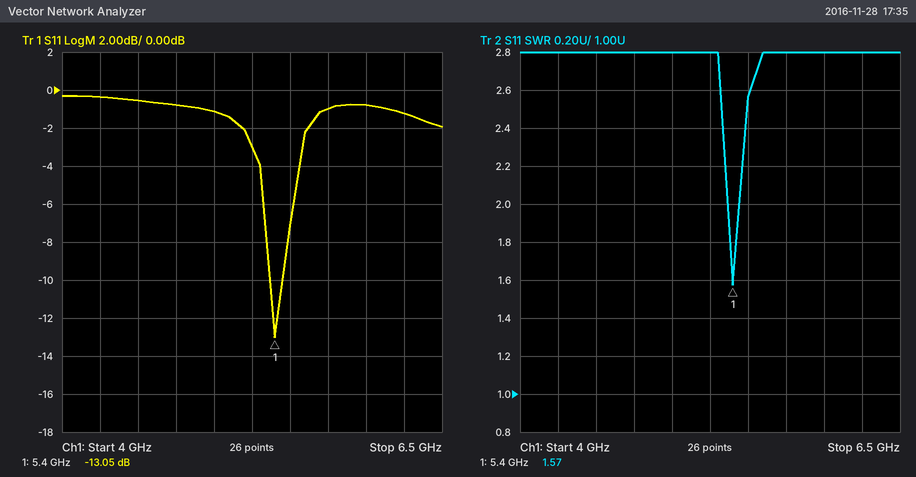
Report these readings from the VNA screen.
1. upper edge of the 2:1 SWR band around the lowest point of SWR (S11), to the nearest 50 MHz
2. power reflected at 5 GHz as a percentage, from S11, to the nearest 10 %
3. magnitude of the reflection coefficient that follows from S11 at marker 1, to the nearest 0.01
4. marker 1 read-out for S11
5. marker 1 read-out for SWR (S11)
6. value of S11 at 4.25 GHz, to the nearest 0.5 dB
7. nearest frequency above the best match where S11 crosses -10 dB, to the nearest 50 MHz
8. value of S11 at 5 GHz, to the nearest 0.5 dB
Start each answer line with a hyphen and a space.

- 5.45 GHz
- 80 %
- 0.22
- -13.05 dB
- 1.57
- -0.5 dB
- 5.45 GHz
- -1.0 dB
